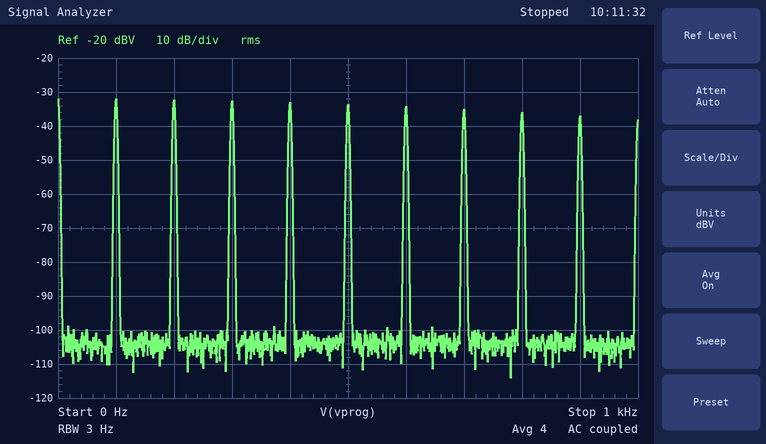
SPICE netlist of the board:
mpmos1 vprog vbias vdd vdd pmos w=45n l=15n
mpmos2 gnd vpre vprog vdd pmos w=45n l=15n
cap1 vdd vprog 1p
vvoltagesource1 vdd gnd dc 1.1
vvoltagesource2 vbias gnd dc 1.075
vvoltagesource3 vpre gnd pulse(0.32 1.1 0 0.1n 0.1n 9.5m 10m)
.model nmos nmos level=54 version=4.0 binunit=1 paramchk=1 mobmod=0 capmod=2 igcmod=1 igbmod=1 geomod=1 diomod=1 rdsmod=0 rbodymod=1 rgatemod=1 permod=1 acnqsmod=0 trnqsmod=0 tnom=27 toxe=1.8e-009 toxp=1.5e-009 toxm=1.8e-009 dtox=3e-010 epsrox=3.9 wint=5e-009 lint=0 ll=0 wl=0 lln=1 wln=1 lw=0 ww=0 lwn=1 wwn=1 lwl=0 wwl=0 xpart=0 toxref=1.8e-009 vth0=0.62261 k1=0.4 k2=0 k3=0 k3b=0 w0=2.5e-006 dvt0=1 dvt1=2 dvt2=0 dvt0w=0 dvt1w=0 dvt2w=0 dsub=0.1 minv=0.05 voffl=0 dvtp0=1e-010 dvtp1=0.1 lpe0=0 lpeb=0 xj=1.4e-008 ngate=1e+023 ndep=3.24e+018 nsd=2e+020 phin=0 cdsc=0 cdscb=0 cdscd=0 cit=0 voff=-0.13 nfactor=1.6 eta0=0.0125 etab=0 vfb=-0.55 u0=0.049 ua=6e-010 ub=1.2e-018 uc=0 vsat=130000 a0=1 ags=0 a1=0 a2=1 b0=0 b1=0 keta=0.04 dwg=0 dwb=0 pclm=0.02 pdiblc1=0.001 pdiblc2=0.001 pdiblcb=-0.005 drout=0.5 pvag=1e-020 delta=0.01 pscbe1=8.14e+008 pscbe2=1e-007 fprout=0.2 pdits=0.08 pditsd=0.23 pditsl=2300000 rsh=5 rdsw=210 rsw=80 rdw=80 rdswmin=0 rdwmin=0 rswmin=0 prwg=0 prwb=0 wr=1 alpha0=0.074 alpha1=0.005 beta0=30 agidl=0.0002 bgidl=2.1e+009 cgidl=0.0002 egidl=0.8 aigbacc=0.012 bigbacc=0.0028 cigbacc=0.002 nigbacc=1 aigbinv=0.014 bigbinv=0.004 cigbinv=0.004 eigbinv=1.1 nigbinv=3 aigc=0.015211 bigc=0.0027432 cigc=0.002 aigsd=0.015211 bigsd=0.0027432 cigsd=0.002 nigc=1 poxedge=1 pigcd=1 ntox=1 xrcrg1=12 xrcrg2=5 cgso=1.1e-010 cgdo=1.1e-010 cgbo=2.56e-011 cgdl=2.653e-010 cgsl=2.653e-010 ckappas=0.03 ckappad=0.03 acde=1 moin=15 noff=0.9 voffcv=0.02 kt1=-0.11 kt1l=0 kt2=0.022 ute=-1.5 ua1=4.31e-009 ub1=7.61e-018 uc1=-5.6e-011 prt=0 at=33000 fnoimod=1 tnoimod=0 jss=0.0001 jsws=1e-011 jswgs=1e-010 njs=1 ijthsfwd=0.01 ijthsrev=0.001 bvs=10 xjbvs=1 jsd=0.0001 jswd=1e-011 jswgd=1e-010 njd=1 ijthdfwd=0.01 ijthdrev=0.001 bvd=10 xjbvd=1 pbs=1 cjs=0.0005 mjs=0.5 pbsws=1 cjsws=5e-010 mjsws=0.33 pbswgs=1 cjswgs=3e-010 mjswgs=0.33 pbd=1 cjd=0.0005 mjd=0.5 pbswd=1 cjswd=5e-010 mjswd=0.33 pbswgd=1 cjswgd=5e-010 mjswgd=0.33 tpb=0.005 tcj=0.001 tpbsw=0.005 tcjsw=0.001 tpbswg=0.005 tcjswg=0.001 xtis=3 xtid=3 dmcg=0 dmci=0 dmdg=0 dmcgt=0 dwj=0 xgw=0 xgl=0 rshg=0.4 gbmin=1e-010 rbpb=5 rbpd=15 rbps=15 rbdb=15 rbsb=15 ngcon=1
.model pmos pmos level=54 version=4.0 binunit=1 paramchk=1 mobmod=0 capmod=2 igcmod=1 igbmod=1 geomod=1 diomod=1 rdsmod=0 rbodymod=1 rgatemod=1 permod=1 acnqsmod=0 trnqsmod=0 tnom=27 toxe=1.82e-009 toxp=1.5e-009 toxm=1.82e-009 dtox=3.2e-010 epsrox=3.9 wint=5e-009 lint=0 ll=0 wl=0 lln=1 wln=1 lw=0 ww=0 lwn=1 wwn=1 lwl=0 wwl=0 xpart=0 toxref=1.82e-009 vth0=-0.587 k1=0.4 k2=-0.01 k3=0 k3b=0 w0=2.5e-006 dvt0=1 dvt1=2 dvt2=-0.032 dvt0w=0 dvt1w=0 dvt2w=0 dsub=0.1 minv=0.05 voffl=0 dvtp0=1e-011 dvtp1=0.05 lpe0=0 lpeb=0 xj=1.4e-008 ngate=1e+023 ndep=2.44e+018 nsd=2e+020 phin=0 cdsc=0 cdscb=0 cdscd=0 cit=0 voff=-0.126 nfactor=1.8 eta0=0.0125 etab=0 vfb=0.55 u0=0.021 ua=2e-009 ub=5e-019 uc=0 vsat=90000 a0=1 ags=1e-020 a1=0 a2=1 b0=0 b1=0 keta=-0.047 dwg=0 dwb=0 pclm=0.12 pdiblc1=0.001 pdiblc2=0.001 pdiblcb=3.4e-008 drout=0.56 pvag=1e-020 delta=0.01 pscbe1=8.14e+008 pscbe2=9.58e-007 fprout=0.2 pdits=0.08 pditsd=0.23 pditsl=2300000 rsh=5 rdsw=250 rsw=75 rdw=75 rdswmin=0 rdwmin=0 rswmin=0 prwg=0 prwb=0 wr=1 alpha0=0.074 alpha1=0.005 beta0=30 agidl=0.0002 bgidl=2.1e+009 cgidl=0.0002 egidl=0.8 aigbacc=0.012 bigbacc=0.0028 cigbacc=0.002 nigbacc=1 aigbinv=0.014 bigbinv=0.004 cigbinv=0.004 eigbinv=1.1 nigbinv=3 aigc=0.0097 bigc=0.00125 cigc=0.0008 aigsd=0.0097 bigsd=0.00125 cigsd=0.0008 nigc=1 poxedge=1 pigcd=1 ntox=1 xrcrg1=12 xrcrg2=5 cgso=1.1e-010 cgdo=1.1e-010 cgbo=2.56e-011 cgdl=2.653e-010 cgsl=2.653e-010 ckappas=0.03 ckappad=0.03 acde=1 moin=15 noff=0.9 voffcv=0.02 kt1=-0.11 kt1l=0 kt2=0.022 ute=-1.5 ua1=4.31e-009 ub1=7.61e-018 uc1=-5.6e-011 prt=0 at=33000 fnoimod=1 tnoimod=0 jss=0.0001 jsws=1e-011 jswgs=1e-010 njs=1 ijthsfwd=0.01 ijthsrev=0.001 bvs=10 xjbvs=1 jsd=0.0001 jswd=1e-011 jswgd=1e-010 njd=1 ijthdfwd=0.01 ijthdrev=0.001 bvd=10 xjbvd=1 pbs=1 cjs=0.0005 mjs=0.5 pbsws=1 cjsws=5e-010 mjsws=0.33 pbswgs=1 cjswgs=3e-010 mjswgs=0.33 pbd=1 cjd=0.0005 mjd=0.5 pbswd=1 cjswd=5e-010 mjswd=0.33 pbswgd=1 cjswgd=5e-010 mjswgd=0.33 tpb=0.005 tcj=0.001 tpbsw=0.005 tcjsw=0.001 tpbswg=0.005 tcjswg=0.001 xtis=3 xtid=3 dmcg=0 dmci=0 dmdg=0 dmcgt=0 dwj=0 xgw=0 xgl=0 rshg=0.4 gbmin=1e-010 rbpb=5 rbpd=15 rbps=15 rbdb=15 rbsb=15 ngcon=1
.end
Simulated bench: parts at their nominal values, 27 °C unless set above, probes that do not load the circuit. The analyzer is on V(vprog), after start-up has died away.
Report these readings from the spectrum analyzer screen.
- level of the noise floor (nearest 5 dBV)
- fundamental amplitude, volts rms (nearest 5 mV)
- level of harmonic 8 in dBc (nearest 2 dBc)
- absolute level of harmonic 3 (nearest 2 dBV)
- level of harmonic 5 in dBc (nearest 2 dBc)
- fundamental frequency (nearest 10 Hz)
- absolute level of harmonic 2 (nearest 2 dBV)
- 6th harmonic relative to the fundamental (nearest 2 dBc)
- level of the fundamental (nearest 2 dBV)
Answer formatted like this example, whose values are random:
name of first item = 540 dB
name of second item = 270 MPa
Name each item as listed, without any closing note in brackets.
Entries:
level of the noise floor = -105 dBV
fundamental amplitude, volts rms = 25 mV
level of harmonic 8 in dBc = -4 dBc
absolute level of harmonic 3 = -32 dBV
level of harmonic 5 in dBc = -2 dBc
fundamental frequency = 100 Hz
absolute level of harmonic 2 = -32 dBV
6th harmonic relative to the fundamental = -2 dBc
level of the fundamental = -32 dBV
